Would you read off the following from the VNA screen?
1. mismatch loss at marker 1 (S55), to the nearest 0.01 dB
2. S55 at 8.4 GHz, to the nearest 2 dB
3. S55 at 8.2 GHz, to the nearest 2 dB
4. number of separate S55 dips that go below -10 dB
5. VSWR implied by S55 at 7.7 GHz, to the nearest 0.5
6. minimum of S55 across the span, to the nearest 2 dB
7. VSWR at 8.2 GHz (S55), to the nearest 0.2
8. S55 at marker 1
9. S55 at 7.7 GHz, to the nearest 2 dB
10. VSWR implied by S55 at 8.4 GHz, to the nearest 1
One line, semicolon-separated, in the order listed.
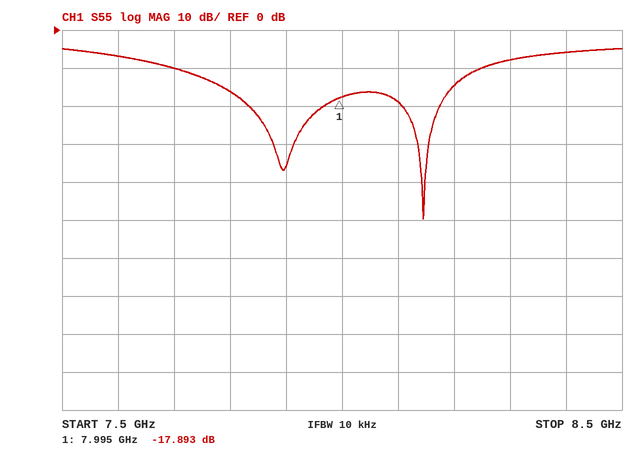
0.07 dB; -6 dB; -14 dB; 2; 2.0; -50 dB; 1.4; -17.893 dB; -10 dB; 3
